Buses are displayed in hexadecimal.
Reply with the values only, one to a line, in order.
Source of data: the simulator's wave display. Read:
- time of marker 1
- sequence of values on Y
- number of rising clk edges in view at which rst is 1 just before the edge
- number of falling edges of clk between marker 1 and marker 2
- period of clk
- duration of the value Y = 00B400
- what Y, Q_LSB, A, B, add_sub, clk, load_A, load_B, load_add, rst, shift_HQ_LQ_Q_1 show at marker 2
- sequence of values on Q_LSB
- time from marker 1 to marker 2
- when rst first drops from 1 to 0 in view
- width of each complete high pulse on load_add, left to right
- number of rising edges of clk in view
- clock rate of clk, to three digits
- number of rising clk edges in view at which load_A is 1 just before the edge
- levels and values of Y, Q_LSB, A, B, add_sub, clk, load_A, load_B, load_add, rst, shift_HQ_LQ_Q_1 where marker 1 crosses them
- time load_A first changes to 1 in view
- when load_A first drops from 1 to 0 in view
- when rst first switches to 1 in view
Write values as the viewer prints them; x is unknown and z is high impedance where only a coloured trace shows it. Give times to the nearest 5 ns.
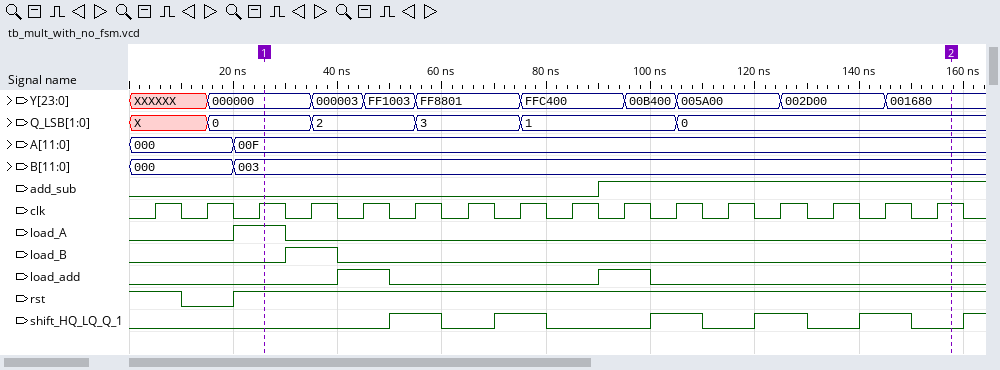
25 ns
XXXXXX, 000000, 000003, FF1003, FF8801, FFC400, 00B400, 005A00, 002D00, 001680
15
13
10 ns
10 ns
Y=001680, Q_LSB=0, A=00F, B=003, add_sub=1, clk=1, load_A=0, load_B=0, load_add=0, rst=1, shift_HQ_LQ_Q_1=0
X, 0, 2, 3, 1, 0
130 ns
10 ns
10 ns, 10 ns
16
100 MHz
1
Y=000000, Q_LSB=0, A=00F, B=003, add_sub=0, clk=1, load_A=1, load_B=0, load_add=0, rst=1, shift_HQ_LQ_Q_1=0
20 ns
30 ns
20 ns
